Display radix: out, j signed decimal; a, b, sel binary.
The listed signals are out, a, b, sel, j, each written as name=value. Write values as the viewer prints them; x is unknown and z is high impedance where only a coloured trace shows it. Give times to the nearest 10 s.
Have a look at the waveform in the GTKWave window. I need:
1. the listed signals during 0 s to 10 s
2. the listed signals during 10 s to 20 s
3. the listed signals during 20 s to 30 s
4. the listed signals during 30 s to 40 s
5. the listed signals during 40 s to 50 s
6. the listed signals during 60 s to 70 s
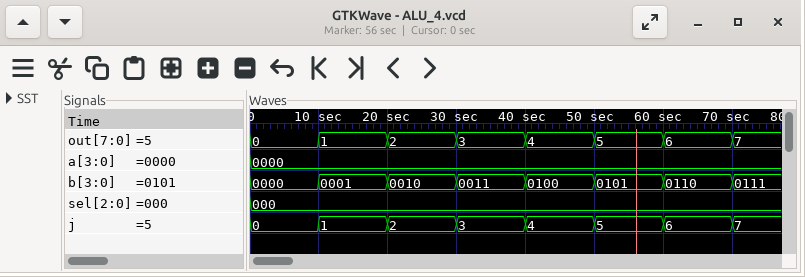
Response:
out=0, a=0000, b=0000, sel=000, j=0
out=1, a=0000, b=0001, sel=000, j=1
out=2, a=0000, b=0010, sel=000, j=2
out=3, a=0000, b=0011, sel=000, j=3
out=4, a=0000, b=0100, sel=000, j=4
out=6, a=0000, b=0110, sel=000, j=6
